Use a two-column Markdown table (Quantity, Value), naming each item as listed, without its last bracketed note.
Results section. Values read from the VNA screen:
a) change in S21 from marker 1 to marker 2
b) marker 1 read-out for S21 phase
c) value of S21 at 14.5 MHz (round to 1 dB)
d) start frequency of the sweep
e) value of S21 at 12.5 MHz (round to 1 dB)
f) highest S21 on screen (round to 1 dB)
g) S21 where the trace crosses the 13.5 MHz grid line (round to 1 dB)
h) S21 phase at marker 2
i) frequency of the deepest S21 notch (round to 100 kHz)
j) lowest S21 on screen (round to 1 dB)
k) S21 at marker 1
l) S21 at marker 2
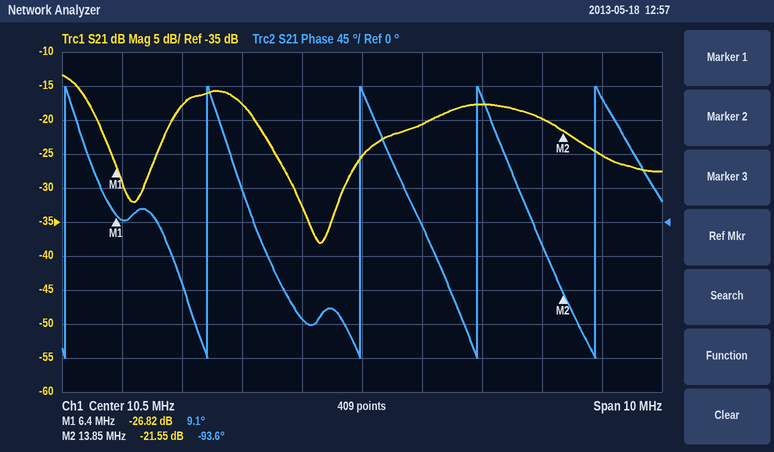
| Quantity | Value |
|---|---|
| change in S21 from marker 1 to marker 2 | 5.27 dB |
| marker 1 read-out for S21 phase | 9.1° |
| value of S21 at 14.5 MHz | -25 dB |
| start frequency of the sweep | 5.5 MHz |
| value of S21 at 12.5 MHz | -18 dB |
| highest S21 on screen | -13 dB |
| S21 where the trace crosses the 13.5 MHz grid line | -20 dB |
| S21 phase at marker 2 | -93.6° |
| frequency of the deepest S21 notch | 9.8 MHz |
| lowest S21 on screen | -38 dB |
| S21 at marker 1 | -26.82 dB |
| S21 at marker 2 | -21.55 dB |
